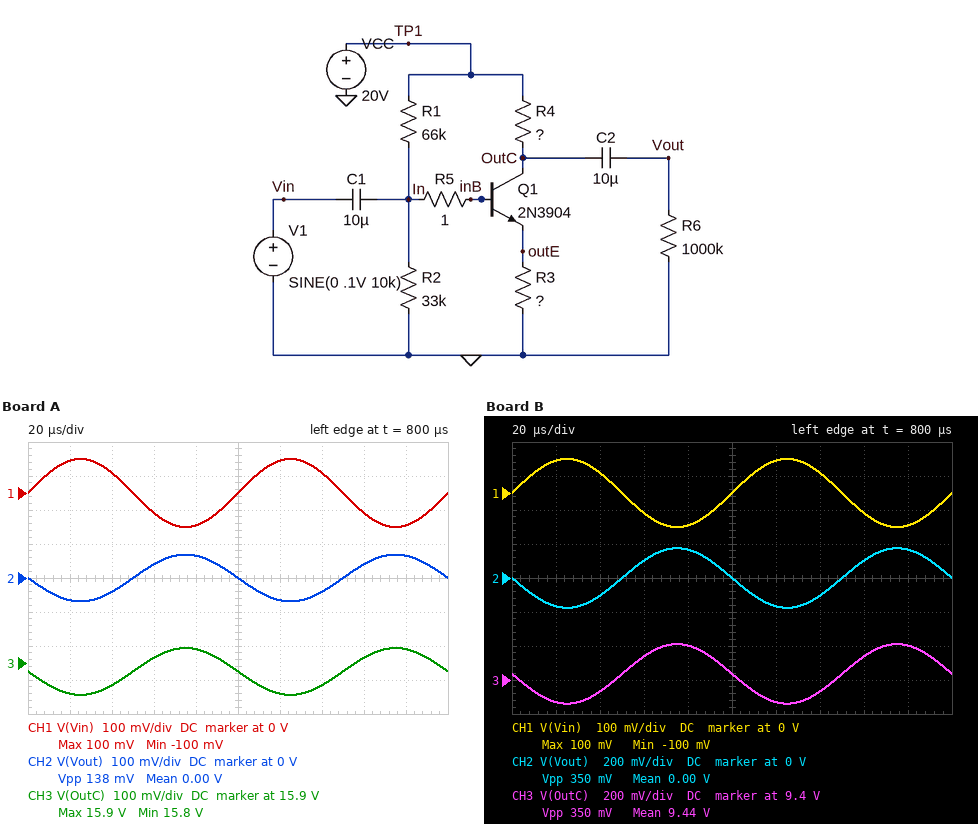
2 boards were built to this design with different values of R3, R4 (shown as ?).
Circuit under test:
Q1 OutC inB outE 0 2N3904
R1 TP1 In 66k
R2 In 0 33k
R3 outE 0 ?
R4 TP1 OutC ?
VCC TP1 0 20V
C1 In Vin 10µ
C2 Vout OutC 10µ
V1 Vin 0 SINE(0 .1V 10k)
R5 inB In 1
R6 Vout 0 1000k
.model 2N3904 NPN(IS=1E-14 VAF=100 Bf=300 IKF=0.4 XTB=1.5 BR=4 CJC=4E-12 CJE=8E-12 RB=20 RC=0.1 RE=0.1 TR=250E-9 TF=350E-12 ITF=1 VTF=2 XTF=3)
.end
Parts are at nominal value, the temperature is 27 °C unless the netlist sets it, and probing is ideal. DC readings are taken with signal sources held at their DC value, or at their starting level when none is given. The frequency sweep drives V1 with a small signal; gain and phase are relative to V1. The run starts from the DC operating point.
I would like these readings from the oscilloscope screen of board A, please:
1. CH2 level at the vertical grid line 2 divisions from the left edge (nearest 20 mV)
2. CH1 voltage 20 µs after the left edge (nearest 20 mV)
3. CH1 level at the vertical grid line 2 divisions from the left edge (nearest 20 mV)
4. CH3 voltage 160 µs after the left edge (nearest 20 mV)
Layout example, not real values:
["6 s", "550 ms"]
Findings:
["-40 mV", "100 mV", "60 mV", "15.92 V"]
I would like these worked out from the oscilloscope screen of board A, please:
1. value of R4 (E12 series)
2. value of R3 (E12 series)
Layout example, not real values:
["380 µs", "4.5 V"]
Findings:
["3.9 kΩ", "5.6 kΩ"]
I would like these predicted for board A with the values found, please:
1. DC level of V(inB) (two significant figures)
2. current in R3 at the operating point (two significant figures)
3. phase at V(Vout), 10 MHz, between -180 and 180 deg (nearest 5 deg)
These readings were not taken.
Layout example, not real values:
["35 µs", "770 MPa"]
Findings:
["6.6 V", "1.1 mA", "125 deg"]
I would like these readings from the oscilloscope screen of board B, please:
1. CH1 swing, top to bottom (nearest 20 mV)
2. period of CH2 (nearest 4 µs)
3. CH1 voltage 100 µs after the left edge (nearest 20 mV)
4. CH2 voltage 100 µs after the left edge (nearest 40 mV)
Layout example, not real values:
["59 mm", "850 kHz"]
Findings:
["200 mV", "100 µs", "0 V", "0 V"]
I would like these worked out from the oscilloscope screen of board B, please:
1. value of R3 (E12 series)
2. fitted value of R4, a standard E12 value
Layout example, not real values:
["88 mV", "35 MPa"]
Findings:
["5.6 kΩ", "10 kΩ"]
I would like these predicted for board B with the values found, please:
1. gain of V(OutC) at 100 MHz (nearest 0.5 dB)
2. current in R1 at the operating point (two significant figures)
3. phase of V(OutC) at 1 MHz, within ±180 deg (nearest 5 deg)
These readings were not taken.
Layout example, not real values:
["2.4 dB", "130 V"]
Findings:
["0.5 dB", "200 µA", "165 deg"]
